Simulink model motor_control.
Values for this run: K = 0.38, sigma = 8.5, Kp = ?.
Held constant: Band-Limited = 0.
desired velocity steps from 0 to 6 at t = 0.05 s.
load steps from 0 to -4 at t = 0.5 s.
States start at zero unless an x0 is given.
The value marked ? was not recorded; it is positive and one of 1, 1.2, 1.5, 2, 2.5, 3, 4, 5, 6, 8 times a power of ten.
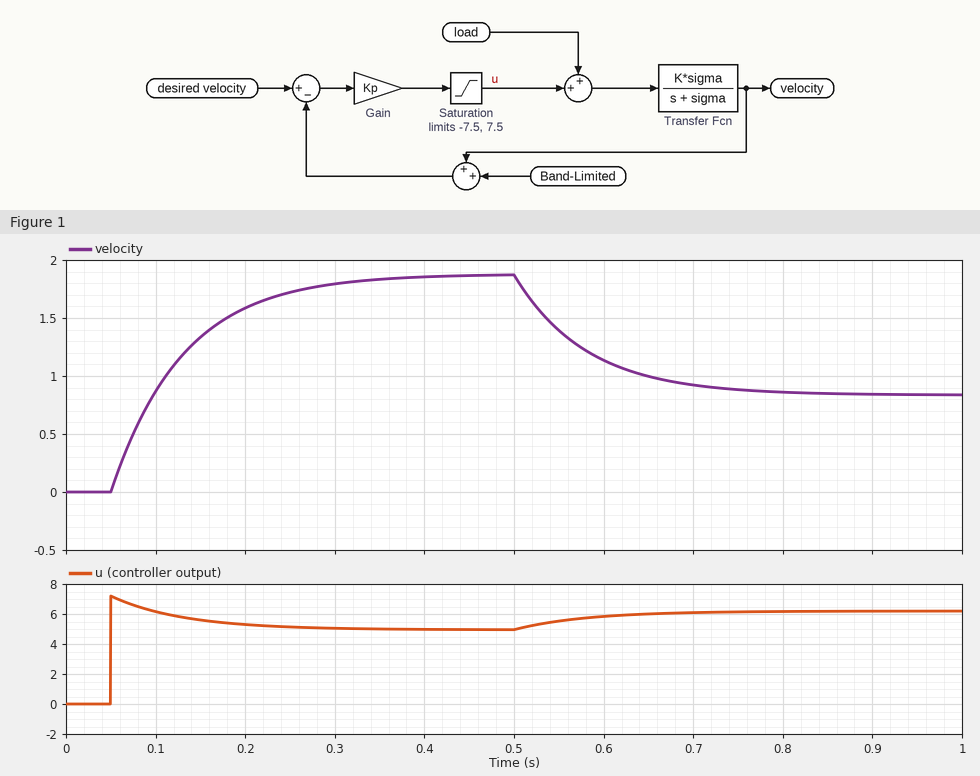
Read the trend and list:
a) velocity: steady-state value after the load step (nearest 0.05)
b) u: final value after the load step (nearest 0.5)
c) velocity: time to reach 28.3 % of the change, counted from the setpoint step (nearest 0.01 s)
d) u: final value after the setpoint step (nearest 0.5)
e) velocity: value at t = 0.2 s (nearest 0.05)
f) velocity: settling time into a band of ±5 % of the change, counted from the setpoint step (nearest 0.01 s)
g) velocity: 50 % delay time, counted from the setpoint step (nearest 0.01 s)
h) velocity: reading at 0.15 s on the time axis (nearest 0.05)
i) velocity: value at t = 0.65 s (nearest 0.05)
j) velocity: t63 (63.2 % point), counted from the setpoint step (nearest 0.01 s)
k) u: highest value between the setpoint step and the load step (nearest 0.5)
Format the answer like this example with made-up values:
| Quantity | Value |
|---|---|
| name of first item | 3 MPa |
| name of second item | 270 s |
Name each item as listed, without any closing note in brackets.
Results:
| Quantity | Value |
|---|---|
| velocity: steady-state value after the load step | 0.85 |
| u: final value after the load step | 6.0 |
| velocity: time to reach 28.3 % of the change, counted from the setpoint step | 0.03 s |
| u: final value after the setpoint step | 5.0 |
| velocity: value at t = 0.2 s | 1.60 |
| velocity: settling time into a band of ±5 % of the change, counted from the setpoint step | 0.24 s |
| velocity: 50 % delay time, counted from the setpoint step | 0.06 s |
| velocity: reading at 0.15 s on the time axis | 1.35 |
| velocity: value at t = 0.65 s | 1.00 |
| velocity: t63 (63.2 % point), counted from the setpoint step | 0.08 s |
| u: highest value between the setpoint step and the load step | 7.0 |
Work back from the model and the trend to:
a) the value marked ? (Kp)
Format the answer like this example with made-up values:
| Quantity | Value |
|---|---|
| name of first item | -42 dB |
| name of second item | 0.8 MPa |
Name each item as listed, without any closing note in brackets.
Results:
| Quantity | Value |
|---|---|
| the value marked ? | 1.2 |
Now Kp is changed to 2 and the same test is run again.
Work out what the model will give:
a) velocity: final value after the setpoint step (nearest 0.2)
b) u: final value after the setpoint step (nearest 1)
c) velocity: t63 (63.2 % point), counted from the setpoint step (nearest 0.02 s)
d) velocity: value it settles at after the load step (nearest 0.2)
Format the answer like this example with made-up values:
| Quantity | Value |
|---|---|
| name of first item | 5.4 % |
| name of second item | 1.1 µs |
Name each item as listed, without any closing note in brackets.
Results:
| Quantity | Value |
|---|---|
| velocity: final value after the setpoint step | 2.6 |
| u: final value after the setpoint step | 7 |
| velocity: t63 (63.2 % point), counted from the setpoint step | 0.10 s |
| velocity: value it settles at after the load step | 1.4 |
